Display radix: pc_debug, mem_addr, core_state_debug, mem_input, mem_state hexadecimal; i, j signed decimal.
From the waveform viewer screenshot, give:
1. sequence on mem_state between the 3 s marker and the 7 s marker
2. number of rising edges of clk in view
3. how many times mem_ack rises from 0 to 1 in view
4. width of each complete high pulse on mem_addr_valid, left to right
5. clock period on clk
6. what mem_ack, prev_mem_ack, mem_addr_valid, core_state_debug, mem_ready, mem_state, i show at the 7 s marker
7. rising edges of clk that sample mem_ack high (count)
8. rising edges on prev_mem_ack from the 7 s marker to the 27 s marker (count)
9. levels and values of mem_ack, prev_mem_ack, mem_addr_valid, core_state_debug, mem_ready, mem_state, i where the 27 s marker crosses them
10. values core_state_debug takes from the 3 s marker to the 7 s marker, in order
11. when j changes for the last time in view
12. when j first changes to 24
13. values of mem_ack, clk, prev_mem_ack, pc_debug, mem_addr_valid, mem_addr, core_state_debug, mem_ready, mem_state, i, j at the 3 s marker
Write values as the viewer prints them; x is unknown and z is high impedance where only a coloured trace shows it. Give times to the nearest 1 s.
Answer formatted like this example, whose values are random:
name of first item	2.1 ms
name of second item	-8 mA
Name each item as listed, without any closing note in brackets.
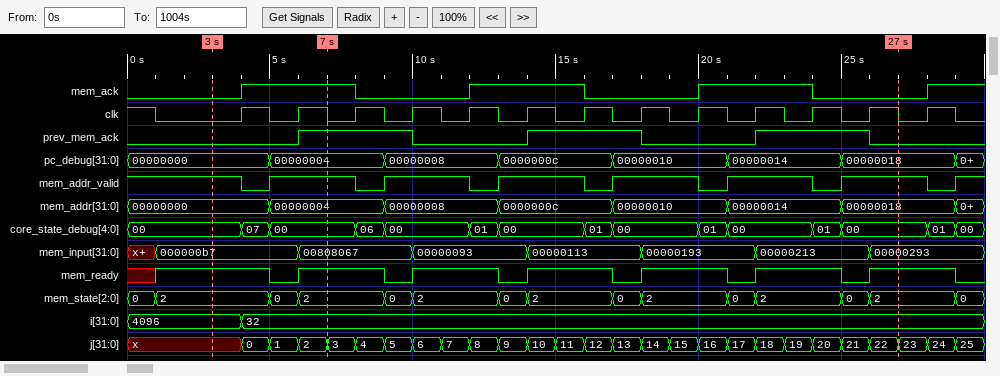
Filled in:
sequence on mem_state between the 3 s marker and the 7 s marker	2, 0, 2
number of rising edges of clk in view	13
how many times mem_ack rises from 0 to 1 in view	4
width of each complete high pulse on mem_addr_valid, left to right	3 s, 3 s, 3 s, 3 s, 3 s, 3 s
clock period on clk	2 s
what mem_ack, prev_mem_ack, mem_addr_valid, core_state_debug, mem_ready, mem_state, i show at the 7 s marker	mem_ack=1, prev_mem_ack=1, mem_addr_valid=1, core_state_debug=00, mem_ready=1, mem_state=2, i=32
rising edges of clk that sample mem_ack high	6
rising edges on prev_mem_ack from the 7 s marker to the 27 s marker	2
levels and values of mem_ack, prev_mem_ack, mem_addr_valid, core_state_debug, mem_ready, mem_state, i where the 27 s marker crosses them	mem_ack=0, prev_mem_ack=0, mem_addr_valid=1, core_state_debug=00, mem_ready=1, mem_state=2, i=32
values core_state_debug takes from the 3 s marker to the 7 s marker, in order	00, 07, 00
when j changes for the last time in view	29 s
when j first changes to 24	28 s
values of mem_ack, clk, prev_mem_ack, pc_debug, mem_addr_valid, mem_addr, core_state_debug, mem_ready, mem_state, i, j at the 3 s marker	mem_ack=0, clk=0, prev_mem_ack=0, pc_debug=00000000, mem_addr_valid=1, mem_addr=00000000, core_state_debug=00, mem_ready=1, mem_state=2, i=4096, j=x
